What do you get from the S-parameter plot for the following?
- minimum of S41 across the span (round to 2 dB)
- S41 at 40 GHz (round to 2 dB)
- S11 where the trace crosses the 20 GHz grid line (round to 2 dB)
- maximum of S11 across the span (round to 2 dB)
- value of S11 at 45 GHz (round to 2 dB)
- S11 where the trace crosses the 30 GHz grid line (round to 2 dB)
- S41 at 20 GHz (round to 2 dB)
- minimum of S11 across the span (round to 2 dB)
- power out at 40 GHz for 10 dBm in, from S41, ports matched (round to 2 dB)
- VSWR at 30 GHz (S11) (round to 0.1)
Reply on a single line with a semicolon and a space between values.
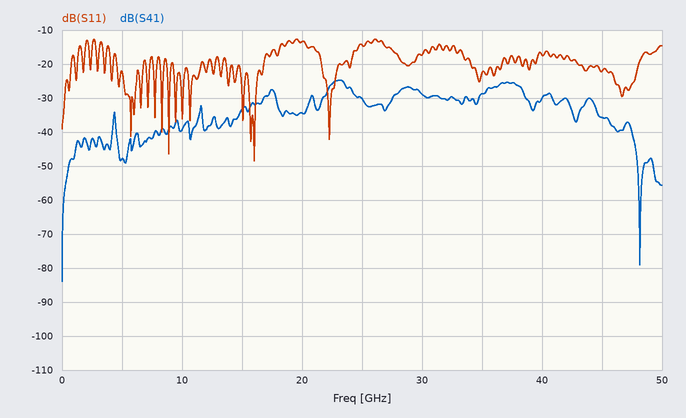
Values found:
-84 dB; -30 dB; -14 dB; -12 dB; -22 dB; -18 dB; -34 dB; -48 dB; -20 dBm; 1.3
